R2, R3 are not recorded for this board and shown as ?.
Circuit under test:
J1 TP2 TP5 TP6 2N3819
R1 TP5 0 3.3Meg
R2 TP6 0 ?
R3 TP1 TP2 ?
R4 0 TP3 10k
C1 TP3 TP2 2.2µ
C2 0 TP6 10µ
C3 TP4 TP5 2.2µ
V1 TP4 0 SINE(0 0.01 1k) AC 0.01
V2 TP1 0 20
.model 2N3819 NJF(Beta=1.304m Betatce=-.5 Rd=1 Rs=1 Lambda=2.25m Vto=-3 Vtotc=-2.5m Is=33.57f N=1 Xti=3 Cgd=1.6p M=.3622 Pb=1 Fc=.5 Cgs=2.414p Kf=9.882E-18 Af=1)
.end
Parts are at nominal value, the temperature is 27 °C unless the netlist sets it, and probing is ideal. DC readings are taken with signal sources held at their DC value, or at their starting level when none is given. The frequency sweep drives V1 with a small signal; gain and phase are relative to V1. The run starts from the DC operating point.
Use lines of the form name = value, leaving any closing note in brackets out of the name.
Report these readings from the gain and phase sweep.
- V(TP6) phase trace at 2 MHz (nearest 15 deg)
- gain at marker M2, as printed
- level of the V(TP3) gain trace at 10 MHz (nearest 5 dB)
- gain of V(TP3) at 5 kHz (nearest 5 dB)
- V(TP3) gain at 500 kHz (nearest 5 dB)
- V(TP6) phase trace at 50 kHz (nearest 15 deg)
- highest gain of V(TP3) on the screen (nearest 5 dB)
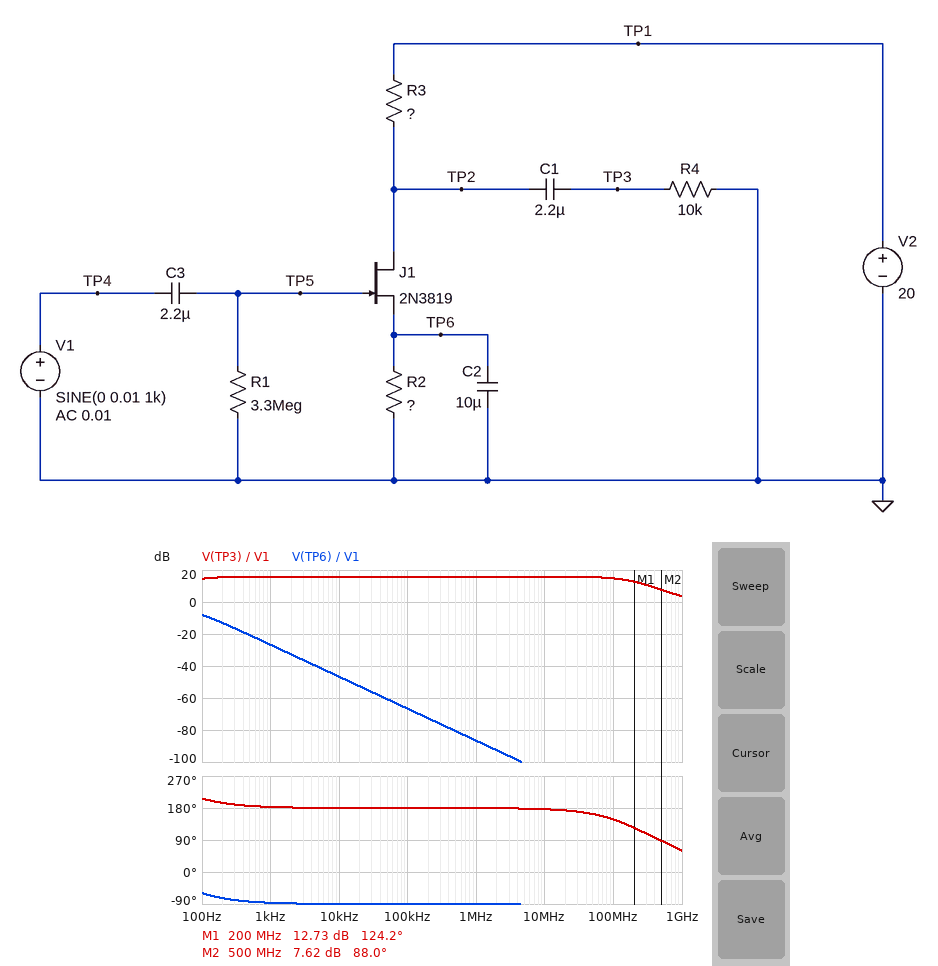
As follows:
V(TP6) phase trace at 2 MHz = -90 deg
gain at marker M2, as printed = 7.62 dB
level of the V(TP3) gain trace at 10 MHz = 15 dB
gain of V(TP3) at 5 kHz = 15 dB
V(TP3) gain at 500 kHz = 15 dB
V(TP6) phase trace at 50 kHz = -90 deg
highest gain of V(TP3) on the screen = 15 dB
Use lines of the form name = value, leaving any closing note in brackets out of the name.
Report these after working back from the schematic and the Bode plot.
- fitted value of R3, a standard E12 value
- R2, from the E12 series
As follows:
fitted value of R3, a standard E12 value = 2.7 kΩ
R2, from the E12 series = 1.2 kΩ
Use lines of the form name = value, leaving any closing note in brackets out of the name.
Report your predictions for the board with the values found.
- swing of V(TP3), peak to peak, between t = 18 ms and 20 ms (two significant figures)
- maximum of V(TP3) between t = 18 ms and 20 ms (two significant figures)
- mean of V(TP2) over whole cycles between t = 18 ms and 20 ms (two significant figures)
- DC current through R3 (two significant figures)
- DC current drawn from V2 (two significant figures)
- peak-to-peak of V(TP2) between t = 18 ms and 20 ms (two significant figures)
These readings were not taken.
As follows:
swing of V(TP3), peak to peak, between t = 18 ms and 20 ms = 120 mV
maximum of V(TP3) between t = 18 ms and 20 ms = 61 mV
mean of V(TP2) over whole cycles between t = 18 ms and 20 ms = 16 V
DC current through R3 = 1.6 mA
DC current drawn from V2 = 1.6 mA
peak-to-peak of V(TP2) between t = 18 ms and 20 ms = 120 mV
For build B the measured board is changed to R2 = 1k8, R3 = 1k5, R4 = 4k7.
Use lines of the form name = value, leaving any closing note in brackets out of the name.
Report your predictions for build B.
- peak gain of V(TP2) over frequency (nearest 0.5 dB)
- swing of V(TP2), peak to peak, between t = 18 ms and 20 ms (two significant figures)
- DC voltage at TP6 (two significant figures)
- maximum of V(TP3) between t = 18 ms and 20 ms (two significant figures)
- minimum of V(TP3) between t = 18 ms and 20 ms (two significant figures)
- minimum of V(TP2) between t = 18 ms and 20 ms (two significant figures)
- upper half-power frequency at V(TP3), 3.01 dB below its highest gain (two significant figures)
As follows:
peak gain of V(TP2) over frequency = 9.0 dB
swing of V(TP2), peak to peak, between t = 18 ms and 20 ms = 56 mV
DC voltage at TP6 = 2.1 V
maximum of V(TP3) between t = 18 ms and 20 ms = 28 mV
minimum of V(TP3) between t = 18 ms and 20 ms = -28 mV
minimum of V(TP2) between t = 18 ms and 20 ms = 18 V
upper half-power frequency at V(TP3), 3.01 dB below its highest gain = 450 MHz
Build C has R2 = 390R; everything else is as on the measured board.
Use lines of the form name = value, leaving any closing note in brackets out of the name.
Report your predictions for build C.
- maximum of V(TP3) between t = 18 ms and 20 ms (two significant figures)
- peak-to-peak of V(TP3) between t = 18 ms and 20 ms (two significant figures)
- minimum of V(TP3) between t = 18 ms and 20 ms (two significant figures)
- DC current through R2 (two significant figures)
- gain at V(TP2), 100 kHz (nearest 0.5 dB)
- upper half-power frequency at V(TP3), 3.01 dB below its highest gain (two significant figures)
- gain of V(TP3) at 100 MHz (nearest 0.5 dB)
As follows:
maximum of V(TP3) between t = 18 ms and 20 ms = 90 mV
peak-to-peak of V(TP3) between t = 18 ms and 20 ms = 180 mV
minimum of V(TP3) between t = 18 ms and 20 ms = -90 mV
DC current through R2 = 3.5 mA
gain at V(TP2), 100 kHz = 19.0 dB
upper half-power frequency at V(TP3), 3.01 dB below its highest gain = 160 MHz
gain of V(TP3) at 100 MHz = 17.5 dB
